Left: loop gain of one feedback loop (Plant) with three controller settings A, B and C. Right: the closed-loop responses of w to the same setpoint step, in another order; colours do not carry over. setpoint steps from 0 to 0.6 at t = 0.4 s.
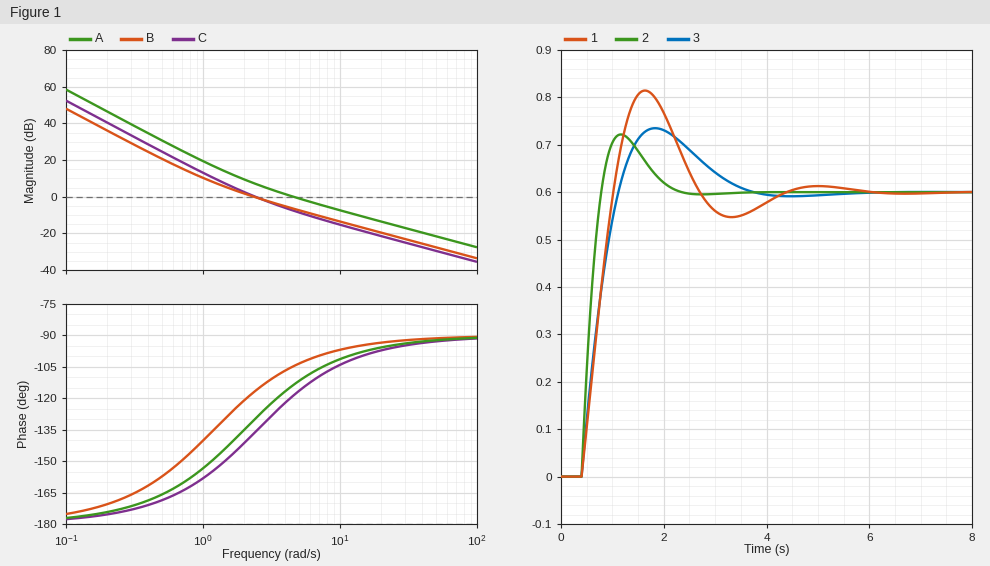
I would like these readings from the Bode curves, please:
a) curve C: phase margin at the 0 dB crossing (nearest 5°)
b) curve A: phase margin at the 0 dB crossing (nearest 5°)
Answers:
45°
65°
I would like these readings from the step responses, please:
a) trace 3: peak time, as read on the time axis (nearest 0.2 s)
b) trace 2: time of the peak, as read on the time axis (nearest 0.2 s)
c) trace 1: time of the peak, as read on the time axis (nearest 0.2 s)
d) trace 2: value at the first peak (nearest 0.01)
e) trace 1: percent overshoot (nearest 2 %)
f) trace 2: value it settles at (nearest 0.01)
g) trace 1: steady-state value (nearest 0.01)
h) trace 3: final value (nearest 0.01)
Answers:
1.8 s
1.2 s
1.6 s
0.72
36 %
0.60
0.60
0.60
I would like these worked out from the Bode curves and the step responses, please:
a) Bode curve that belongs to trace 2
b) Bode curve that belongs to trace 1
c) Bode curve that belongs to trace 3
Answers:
A
C
B
